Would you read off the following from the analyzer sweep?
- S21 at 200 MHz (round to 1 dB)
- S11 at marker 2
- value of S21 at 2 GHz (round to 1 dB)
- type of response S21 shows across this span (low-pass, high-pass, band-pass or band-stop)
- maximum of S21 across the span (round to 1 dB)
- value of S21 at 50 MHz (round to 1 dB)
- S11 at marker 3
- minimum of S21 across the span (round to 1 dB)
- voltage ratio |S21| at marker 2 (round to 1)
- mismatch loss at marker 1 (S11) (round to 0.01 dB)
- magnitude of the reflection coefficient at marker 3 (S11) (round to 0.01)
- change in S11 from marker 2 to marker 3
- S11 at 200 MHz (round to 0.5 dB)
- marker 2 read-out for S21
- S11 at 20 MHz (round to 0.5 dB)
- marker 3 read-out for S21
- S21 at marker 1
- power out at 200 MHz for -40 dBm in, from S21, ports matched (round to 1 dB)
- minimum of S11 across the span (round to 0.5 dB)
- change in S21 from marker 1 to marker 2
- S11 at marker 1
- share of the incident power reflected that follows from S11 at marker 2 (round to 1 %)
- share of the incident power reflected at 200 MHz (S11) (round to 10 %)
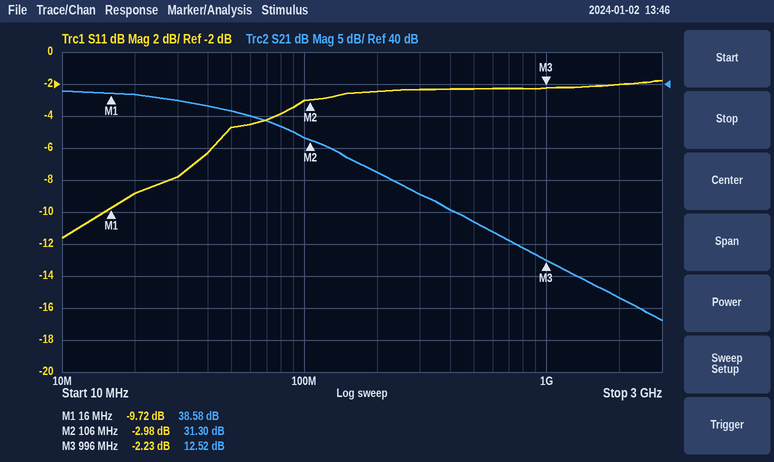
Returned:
26 dB
-2.98 dB
7 dB
low-pass
39 dB
36 dB
-2.23 dB
3 dB
37
0.49 dB
0.77
0.75 dB
-2.5 dB
31.30 dB
-9.0 dB
12.52 dB
38.58 dB
-14 dBm
-11.5 dB
-7.28 dB
-9.72 dB
50 %
60 %
